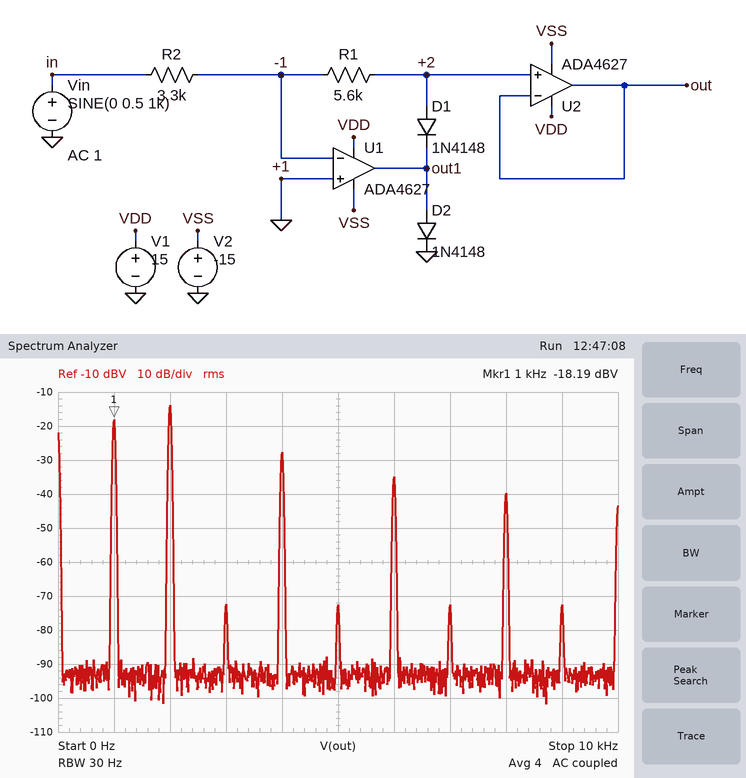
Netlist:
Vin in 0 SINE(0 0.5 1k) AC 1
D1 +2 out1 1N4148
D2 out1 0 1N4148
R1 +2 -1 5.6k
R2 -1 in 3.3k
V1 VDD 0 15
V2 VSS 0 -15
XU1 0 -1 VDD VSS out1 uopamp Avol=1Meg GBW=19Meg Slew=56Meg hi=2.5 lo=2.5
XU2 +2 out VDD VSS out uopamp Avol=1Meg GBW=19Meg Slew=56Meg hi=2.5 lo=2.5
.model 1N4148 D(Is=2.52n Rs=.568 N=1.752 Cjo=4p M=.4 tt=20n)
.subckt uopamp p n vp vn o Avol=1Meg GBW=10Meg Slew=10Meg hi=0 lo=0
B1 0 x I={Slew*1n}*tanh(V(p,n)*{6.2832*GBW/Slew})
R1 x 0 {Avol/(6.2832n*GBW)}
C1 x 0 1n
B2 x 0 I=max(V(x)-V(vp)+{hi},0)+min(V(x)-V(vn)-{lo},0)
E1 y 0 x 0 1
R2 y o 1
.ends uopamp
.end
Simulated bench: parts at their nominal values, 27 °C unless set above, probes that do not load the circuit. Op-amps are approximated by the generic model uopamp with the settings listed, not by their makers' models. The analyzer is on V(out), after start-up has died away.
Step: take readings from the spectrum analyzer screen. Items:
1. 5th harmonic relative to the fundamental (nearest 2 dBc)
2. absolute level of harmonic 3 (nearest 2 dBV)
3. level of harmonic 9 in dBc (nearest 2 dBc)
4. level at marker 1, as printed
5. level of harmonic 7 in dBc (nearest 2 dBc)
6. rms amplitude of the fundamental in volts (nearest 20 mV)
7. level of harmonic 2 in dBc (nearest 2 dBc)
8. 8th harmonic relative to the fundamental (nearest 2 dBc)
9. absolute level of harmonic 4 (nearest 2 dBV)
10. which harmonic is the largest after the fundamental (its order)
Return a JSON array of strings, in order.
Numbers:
["-54 dBc", "-72 dBV", "-54 dBc", "-18.19 dBV", "-54 dBc", "120 mV", "4 dBc", "-22 dBc", "-28 dBV", "2"]
